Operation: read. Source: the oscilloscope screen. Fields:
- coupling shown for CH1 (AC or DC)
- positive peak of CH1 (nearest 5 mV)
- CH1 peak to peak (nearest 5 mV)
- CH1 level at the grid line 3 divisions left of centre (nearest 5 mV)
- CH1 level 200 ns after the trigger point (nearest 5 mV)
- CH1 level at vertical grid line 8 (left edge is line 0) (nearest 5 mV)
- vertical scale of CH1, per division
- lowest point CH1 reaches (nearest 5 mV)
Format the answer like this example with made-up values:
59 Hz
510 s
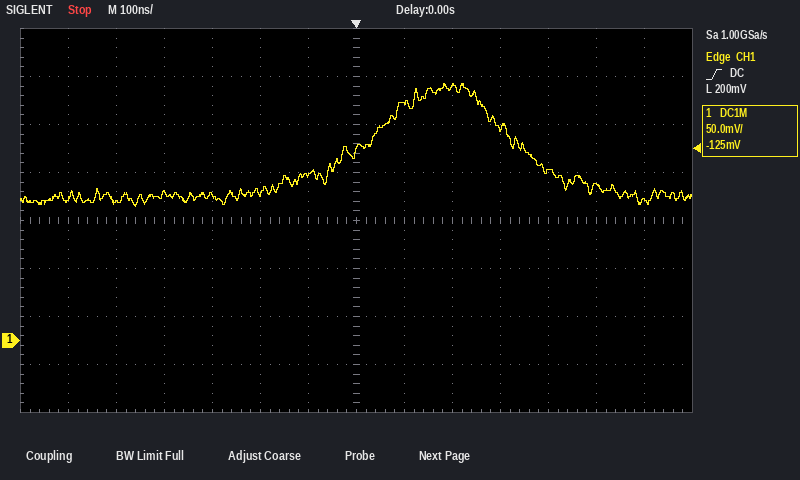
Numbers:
DC
270 mV
130 mV
150 mV
265 mV
250 mV
50 mV
140 mV
